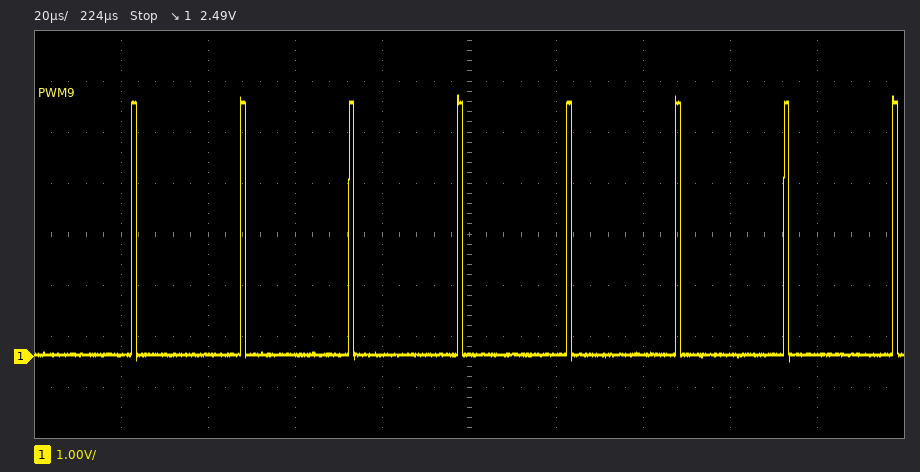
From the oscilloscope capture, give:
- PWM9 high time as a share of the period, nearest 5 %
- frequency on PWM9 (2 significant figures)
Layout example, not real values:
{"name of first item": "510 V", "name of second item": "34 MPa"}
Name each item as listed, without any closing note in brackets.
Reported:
{"PWM9 high time as a share of the period, nearest 5 %": "5 %", "frequency on PWM9": "40 kHz"}
